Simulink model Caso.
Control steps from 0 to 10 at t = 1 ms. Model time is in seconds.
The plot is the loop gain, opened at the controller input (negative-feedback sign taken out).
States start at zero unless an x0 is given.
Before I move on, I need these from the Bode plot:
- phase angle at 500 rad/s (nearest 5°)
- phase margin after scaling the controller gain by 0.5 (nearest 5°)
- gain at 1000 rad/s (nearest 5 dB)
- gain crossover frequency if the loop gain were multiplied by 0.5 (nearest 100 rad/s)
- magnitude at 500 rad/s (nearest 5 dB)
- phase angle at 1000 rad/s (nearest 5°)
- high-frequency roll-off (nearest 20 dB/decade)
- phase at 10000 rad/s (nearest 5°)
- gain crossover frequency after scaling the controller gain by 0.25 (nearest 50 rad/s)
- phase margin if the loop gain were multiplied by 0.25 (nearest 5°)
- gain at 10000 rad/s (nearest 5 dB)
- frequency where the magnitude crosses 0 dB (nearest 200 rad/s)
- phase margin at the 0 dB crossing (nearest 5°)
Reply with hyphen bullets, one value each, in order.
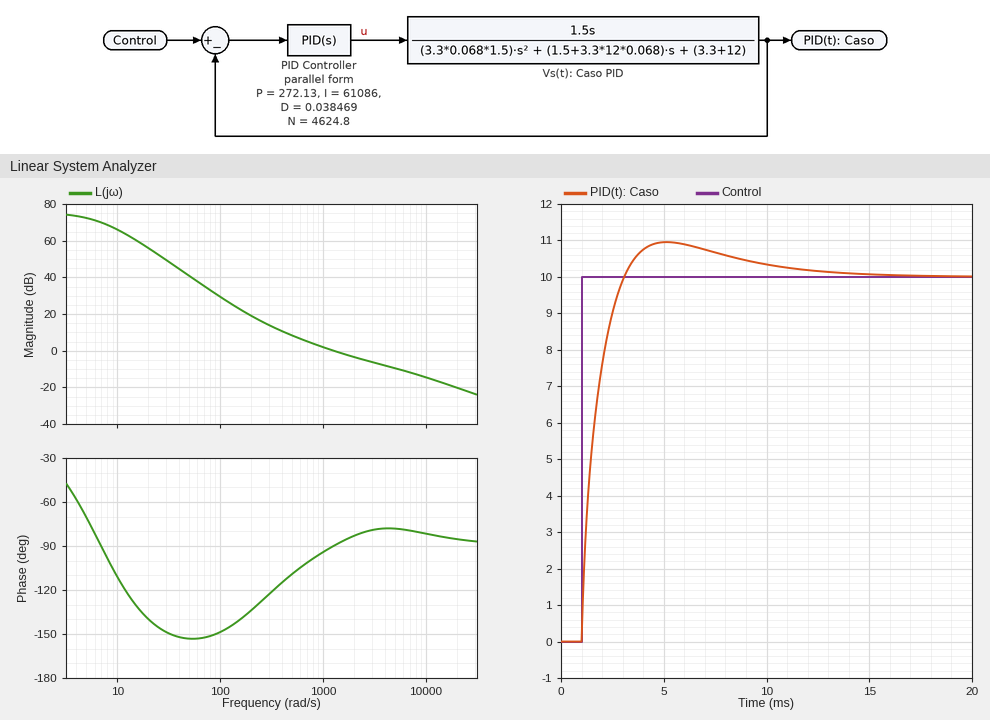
- -110°
- 75°
- 0 dB
- 600 rad/s
- 10 dB
- -95°
- -20 dB/decade
- -80°
- 350 rad/s
- 60°
- -15 dB
- 1200 rad/s
- 90°
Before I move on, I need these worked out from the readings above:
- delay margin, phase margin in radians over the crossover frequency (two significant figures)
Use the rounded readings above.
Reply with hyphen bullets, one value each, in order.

- 0.0013 s
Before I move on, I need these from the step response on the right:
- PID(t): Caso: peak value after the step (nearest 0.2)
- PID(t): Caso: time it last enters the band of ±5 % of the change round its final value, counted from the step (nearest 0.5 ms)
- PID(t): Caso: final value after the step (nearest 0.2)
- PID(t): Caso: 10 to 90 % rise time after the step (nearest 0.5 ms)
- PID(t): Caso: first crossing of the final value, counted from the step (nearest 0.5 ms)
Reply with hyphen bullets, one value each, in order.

- 11.0
- 7.5 ms
- 10.0
- 1.5 ms
- 2.0 ms
